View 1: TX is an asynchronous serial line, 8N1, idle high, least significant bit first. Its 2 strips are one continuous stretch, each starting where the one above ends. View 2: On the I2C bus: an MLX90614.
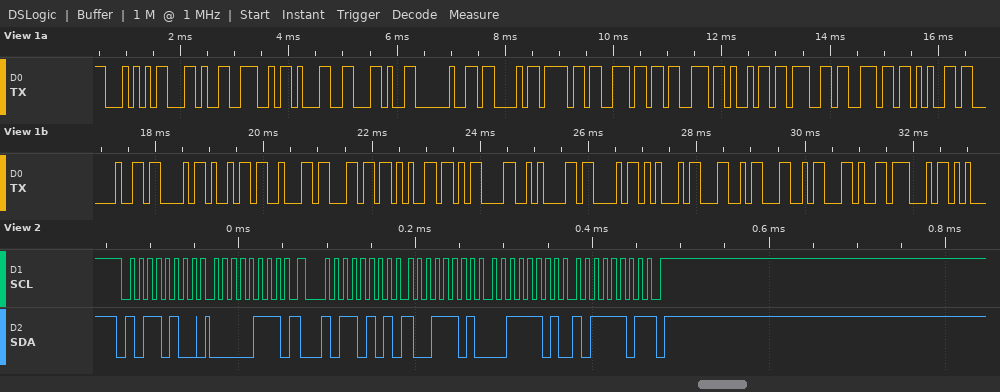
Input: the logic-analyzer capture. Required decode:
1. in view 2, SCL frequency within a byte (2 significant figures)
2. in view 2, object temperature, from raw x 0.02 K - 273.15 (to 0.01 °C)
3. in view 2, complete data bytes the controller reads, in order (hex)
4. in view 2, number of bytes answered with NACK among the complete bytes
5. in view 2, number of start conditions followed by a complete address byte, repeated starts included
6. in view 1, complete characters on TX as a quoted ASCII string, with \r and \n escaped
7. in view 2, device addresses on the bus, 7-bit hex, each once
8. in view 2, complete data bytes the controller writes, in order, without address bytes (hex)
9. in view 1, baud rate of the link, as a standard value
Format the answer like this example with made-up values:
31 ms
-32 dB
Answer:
100 kHz
42.31 °C
9D 3D BD
1
2
"T,N1, Consigne Cible\r\nCELL,G"
0x5A
07
9600 baud
